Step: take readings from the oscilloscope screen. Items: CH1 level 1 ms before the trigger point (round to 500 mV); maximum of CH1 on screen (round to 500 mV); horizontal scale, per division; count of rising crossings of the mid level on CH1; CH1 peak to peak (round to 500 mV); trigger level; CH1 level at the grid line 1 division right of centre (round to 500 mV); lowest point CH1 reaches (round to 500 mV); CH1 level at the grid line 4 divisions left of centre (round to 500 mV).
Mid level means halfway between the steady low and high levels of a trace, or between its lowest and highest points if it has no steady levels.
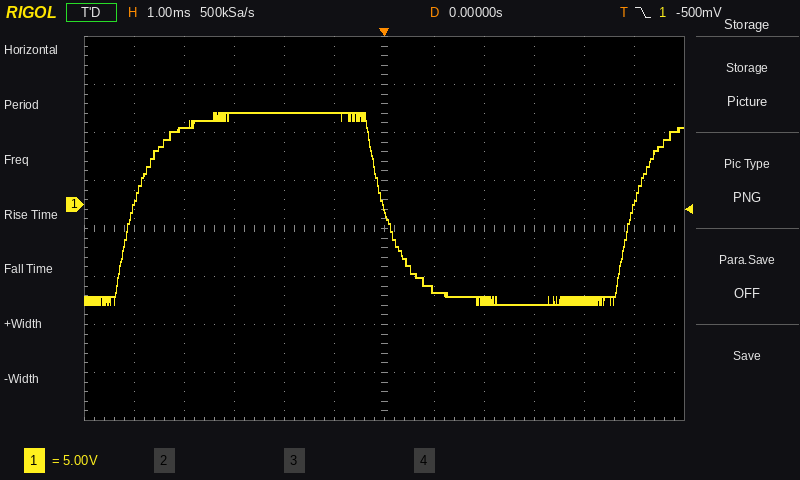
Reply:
9.5 V
9.5 V
1 ms
2
20.0 V
-500 mV
-9.0 V
-10.5 V
8.0 V
